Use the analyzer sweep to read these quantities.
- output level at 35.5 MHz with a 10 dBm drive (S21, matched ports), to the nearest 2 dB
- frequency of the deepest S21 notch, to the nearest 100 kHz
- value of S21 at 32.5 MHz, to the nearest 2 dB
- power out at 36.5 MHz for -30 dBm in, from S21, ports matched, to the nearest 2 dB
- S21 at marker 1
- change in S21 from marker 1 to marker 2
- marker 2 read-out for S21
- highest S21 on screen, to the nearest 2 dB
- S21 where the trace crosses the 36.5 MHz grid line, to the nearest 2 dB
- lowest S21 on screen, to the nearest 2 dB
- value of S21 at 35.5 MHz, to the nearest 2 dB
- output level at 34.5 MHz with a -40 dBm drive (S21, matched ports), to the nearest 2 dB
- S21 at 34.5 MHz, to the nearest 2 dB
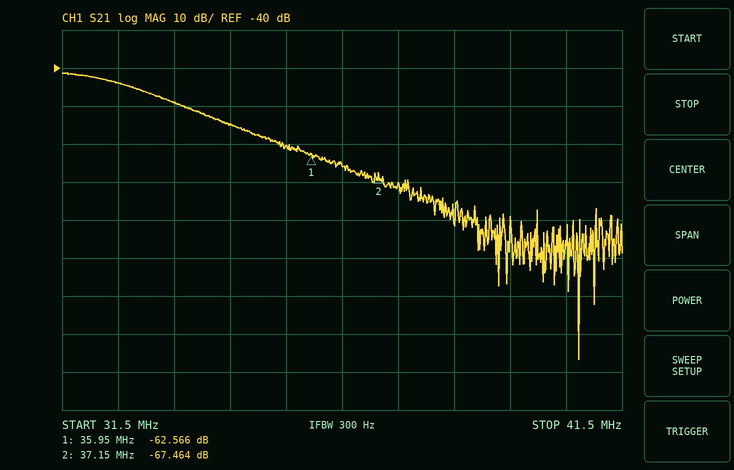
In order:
-50 dBm
40.7 MHz
-44 dB
-96 dBm
-62.566 dB
-4.898 dB
-67.464 dB
-42 dB
-66 dB
-116 dB
-60 dB
-94 dBm
-54 dB
